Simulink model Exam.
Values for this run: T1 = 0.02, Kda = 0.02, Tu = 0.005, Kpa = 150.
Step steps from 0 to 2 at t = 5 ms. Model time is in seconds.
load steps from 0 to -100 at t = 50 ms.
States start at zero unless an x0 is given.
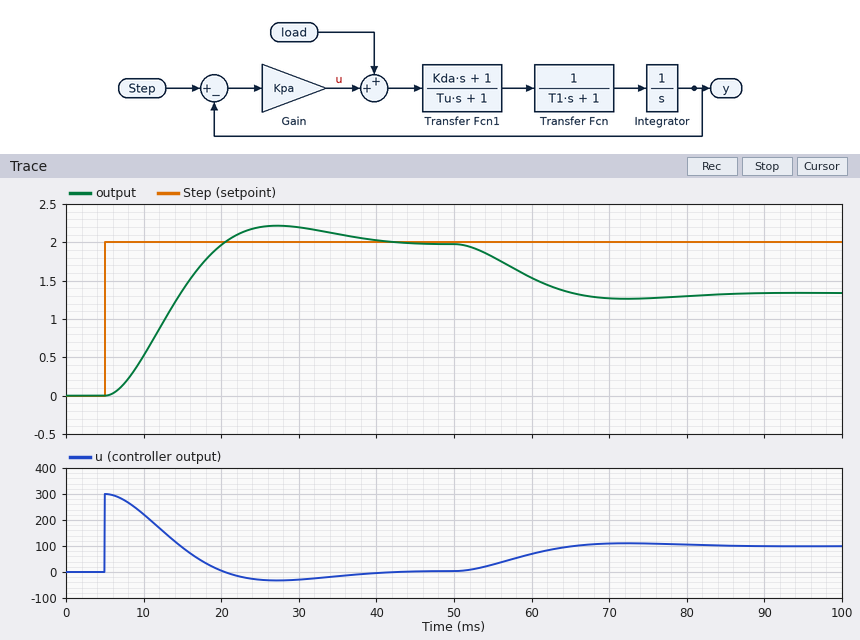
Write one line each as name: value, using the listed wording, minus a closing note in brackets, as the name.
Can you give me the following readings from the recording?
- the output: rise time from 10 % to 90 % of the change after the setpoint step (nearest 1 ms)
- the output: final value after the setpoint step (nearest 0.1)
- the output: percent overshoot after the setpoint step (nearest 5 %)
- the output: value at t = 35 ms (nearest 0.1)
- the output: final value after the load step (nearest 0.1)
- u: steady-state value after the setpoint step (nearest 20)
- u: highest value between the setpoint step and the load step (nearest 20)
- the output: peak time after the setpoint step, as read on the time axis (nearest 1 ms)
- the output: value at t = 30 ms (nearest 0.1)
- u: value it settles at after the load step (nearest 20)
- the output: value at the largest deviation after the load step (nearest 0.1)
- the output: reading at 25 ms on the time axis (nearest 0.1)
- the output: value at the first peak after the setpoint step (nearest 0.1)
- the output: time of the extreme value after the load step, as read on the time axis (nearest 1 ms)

the output: rise time from 10 % to 90 % of the change after the setpoint step: 10 ms
the output: final value after the setpoint step: 2.0
the output: percent overshoot after the setpoint step: 10 %
the output: value at t = 35 ms: 2.1
the output: final value after the load step: 1.3
u: steady-state value after the setpoint step: 0
u: highest value between the setpoint step and the load step: 300
the output: peak time after the setpoint step, as read on the time axis: 27 ms
the output: value at t = 30 ms: 2.2
u: value it settles at after the load step: 100
the output: value at the largest deviation after the load step: 1.3
the output: reading at 25 ms on the time axis: 2.2
the output: value at the first peak after the setpoint step: 2.2
the output: time of the extreme value after the load step, as read on the time axis: 72 ms
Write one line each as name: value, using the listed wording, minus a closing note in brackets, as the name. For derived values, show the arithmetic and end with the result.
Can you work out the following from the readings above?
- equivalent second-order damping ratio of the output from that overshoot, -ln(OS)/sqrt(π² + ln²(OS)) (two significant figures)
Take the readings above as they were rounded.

equivalent second-order damping ratio of the output from that overshoot, -ln(OS)/sqrt(π² + ln²(OS)): ln(0.1) = -2.303; 2.303 / sqrt(9.870 + 5.302) = 0.59
